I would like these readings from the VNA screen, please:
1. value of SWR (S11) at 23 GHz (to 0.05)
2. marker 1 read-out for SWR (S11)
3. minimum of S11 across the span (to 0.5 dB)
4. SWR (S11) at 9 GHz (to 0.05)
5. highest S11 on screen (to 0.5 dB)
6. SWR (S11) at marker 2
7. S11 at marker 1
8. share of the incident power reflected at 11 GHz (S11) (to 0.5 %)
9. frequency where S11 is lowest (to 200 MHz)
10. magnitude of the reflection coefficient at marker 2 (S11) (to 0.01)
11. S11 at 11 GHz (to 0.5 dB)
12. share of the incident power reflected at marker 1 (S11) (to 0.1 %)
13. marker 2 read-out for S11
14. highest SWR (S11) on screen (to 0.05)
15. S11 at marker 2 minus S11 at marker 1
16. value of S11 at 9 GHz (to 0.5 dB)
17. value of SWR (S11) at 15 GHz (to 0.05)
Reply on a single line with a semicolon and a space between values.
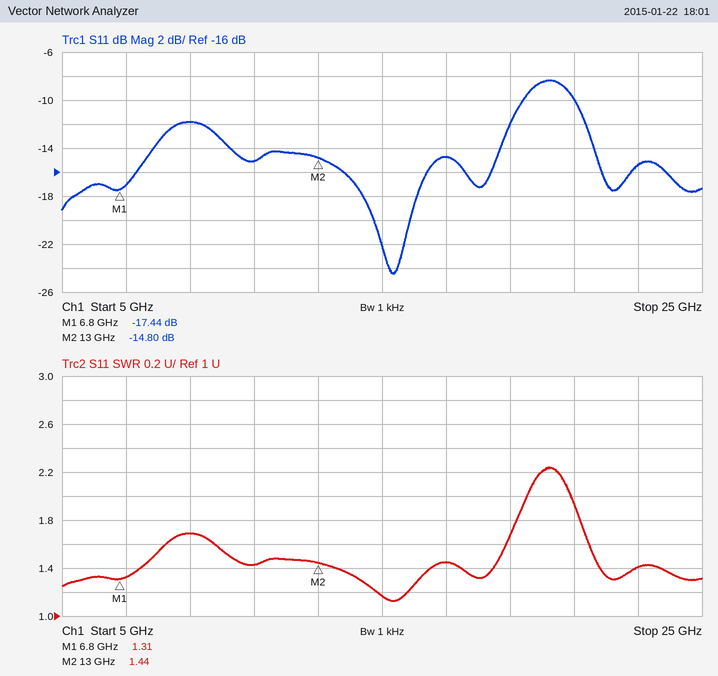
1.40; 1.31; -24.5 dB; 1.70; -8.5 dB; 1.44; -17.44 dB; 3.0 %; 15.4 GHz; 0.18; -15.0 dB; 1.8 %; -14.80 dB; 2.25; 2.64 dB; -12.0 dB; 1.15
